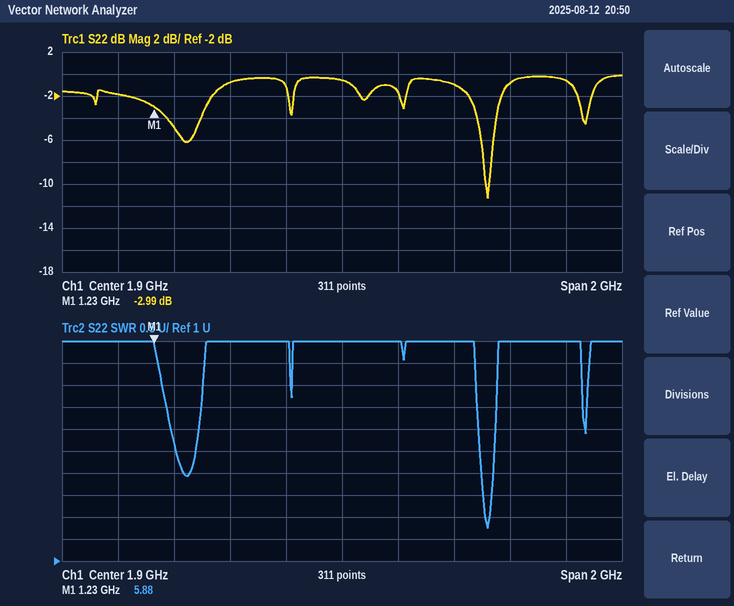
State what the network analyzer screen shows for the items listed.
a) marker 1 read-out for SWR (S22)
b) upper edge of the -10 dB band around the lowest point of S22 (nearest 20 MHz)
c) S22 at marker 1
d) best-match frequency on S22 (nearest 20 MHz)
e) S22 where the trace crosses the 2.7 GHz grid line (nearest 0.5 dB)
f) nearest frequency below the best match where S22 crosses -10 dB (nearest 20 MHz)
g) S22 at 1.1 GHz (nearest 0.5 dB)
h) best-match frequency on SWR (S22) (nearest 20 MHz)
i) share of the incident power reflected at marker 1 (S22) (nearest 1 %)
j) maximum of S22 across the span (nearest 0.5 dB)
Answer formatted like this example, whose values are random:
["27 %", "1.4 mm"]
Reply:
["5.88", "2.42 GHz", "-2.99 dB", "2.42 GHz", "-0.5 dB", "2.42 GHz", "-2.0 dB", "2.42 GHz", "50 %", "0.0 dB"]
